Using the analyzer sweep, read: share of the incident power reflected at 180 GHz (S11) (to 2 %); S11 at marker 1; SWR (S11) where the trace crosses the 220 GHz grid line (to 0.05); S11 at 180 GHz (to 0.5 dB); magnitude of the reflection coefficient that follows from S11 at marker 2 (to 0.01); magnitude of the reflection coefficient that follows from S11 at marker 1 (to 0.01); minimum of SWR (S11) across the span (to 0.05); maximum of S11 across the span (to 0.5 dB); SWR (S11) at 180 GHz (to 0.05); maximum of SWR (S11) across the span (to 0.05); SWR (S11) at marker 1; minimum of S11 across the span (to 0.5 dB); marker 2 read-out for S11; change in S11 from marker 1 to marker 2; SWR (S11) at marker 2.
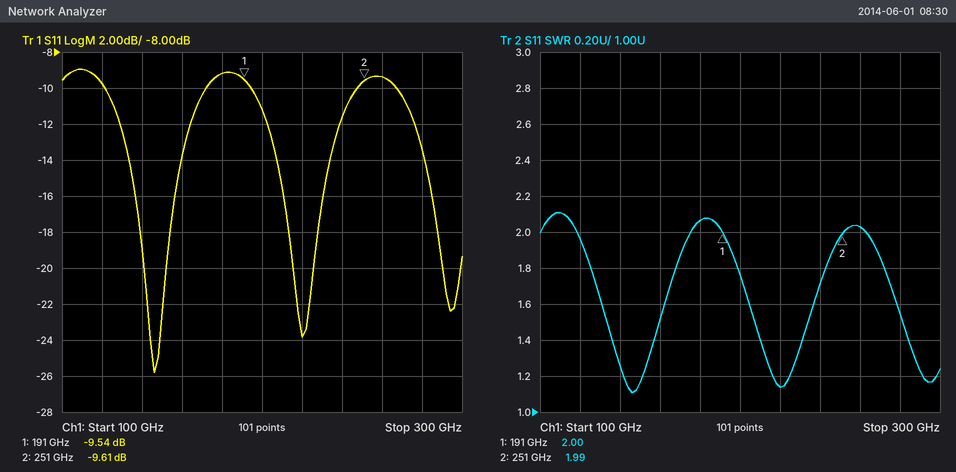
12 %
-9.54 dB
1.15
-9.0 dB
0.33
0.33
1.10
-9.0 dB
2.05
2.10
2.00
-26.0 dB
-9.61 dB
-0.07 dB
1.99
